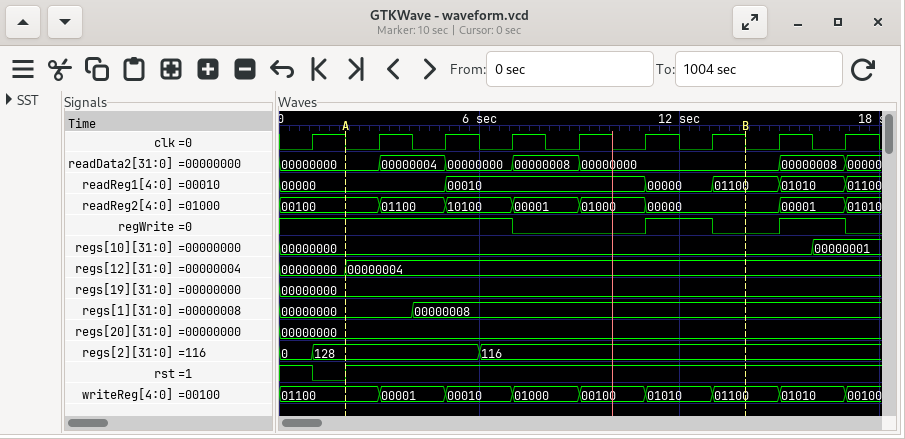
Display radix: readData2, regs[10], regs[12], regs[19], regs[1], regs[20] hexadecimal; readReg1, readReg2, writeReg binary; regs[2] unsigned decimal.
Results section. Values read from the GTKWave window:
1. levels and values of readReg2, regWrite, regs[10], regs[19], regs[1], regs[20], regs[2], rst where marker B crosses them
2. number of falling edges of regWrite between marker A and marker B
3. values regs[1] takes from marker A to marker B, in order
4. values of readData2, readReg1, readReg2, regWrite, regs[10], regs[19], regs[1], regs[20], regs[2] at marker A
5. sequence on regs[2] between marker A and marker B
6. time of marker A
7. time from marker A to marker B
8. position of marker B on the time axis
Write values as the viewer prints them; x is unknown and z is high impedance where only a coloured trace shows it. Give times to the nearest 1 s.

readReg2=00000, regWrite=0, regs[10]=00000000, regs[19]=00000000, regs[1]=00000008, regs[20]=00000000, regs[2]=116, rst=1
2
00000000, 00000008
readData2=00000000, readReg1=00000, readReg2=00100, regWrite=1, regs[10]=00000000, regs[19]=00000000, regs[1]=00000000, regs[20]=00000000, regs[2]=128
128, 116
2 s
12 s
14 s
